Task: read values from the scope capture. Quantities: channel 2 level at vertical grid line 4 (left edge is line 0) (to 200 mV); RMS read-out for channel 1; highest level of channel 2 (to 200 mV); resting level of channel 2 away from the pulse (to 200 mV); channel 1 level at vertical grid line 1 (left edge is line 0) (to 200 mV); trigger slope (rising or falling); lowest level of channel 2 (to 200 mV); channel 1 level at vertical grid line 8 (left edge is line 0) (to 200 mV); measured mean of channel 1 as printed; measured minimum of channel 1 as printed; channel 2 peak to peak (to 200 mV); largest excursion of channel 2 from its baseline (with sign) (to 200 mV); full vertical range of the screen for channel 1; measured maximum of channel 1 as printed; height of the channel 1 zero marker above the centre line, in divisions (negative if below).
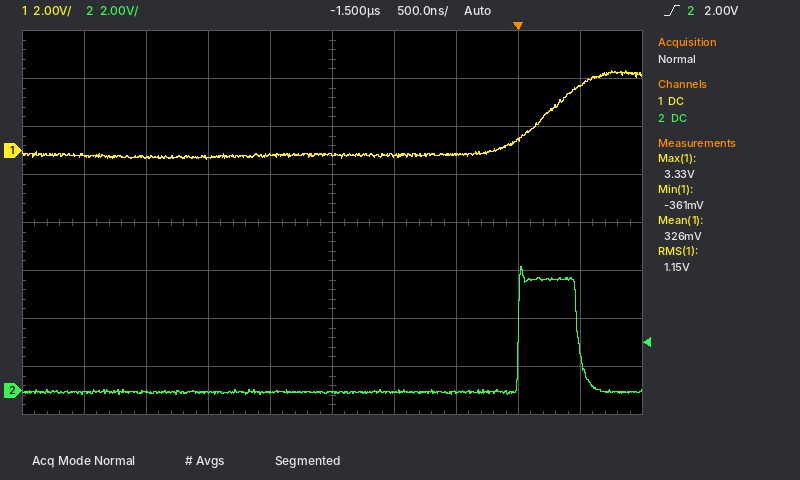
0.0 V
1.15 V
5.2 V
0.0 V
-200 mV
rising
-200 mV
400 mV
326 mV
-361 mV
5.4 V
+5.2 V
16 V
3.33 V
+1.5 div
